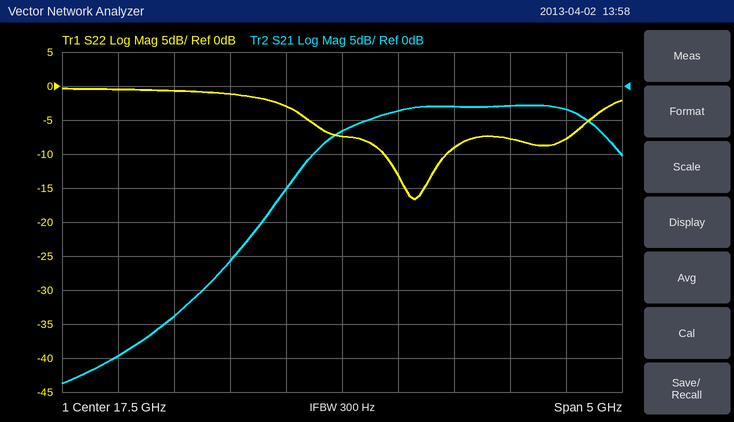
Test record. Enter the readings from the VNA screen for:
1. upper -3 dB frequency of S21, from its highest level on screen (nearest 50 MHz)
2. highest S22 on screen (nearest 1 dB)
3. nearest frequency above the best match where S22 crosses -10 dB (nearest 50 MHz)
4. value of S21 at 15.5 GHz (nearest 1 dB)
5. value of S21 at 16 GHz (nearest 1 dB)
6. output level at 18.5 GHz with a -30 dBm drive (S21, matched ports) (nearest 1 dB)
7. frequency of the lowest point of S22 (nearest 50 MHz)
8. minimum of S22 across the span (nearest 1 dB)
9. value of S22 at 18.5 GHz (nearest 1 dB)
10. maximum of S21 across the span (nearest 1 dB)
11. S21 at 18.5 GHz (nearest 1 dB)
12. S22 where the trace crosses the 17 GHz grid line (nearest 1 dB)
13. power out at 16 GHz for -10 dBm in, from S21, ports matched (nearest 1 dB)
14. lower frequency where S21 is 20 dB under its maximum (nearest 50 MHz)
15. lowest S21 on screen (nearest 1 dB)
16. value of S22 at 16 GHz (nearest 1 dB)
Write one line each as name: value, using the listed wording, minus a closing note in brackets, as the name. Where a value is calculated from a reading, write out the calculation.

upper -3 dB frequency of S21, from its highest level on screen: 19.75 GHz
highest S22 on screen: 0 dB
nearest frequency above the best match where S22 crosses -10 dB: 18.45 GHz
value of S21 at 15.5 GHz: -40 dB
value of S21 at 16 GHz: -34 dB
output level at 18.5 GHz with a -30 dBm drive (S21, matched ports): -30 dBm + (-3 dB) = -33 dBm
frequency of the lowest point of S22: 18.15 GHz
minimum of S22 across the span: -17 dB
value of S22 at 18.5 GHz: -9 dB
maximum of S21 across the span: -3 dB
S21 at 18.5 GHz: -3 dB
S22 where the trace crosses the 17 GHz grid line: -3 dB
power out at 16 GHz for -10 dBm in, from S21, ports matched: -10 dBm + (-34 dB) = -44 dBm
lower frequency where S21 is 20 dB under its maximum: 16.65 GHz
lowest S21 on screen: -44 dB
value of S22 at 16 GHz: -1 dB
